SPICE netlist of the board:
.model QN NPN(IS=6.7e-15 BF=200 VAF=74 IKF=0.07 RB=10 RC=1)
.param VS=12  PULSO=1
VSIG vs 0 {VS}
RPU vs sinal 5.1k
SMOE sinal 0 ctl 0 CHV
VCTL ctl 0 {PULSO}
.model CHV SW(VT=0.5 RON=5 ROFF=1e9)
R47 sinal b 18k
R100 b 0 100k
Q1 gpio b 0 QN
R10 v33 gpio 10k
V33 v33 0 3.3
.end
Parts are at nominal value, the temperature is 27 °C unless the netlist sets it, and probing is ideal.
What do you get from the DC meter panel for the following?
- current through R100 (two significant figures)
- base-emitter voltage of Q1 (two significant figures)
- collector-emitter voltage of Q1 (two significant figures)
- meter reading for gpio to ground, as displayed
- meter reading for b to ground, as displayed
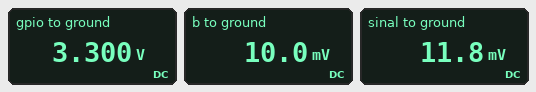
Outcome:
100 nA
10 mV
3.3 V
3.300 V
10.0 mV
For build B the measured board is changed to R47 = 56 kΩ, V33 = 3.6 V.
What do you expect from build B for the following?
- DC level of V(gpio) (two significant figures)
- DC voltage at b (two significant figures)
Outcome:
3.6 V
7.5 mV
